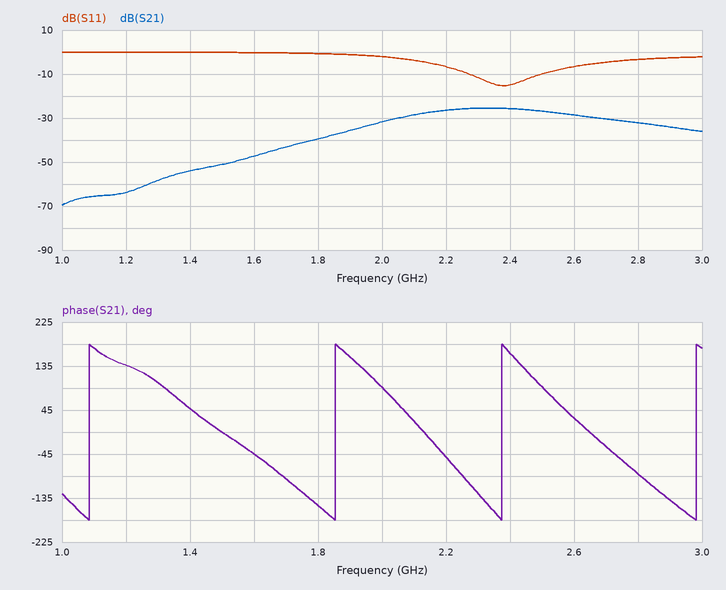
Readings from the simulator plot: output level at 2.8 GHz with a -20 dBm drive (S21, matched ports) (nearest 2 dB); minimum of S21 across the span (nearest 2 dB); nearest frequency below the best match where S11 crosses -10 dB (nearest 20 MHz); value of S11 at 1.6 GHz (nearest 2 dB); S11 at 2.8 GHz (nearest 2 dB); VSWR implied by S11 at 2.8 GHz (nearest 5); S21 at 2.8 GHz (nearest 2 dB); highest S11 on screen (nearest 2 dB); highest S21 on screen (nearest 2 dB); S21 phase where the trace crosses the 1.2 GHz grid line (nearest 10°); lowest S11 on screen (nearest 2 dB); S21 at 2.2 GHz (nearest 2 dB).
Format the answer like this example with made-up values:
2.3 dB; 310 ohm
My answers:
-52 dBm; -70 dB; 2.28 GHz; 0 dB; -4 dB; 5; -32 dB; 0 dB; -26 dB; 140°; -16 dB; -26 dB
